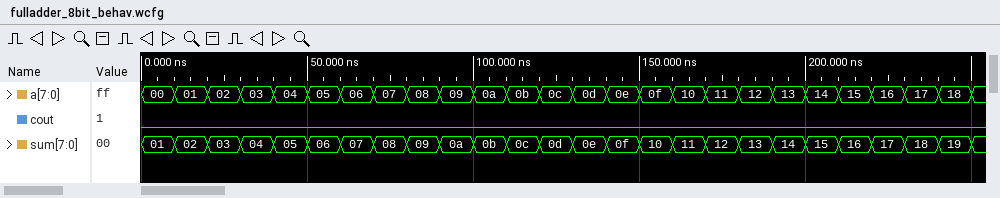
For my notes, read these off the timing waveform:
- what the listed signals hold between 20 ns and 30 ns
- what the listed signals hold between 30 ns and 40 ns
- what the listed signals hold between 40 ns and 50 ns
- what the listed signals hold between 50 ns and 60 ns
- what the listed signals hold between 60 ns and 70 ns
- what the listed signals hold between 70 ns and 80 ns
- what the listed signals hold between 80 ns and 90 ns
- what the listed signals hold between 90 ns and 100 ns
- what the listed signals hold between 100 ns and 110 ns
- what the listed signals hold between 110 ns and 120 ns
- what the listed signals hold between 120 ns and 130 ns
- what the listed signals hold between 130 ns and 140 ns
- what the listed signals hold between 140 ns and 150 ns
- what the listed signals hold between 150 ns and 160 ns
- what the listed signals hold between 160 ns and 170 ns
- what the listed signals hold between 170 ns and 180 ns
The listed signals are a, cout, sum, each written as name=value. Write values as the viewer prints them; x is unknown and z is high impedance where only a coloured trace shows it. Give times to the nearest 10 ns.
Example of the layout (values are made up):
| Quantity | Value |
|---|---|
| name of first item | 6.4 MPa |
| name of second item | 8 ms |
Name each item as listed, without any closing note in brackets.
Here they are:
| Quantity | Value |
|---|---|
| what the listed signals hold between 20 ns and 30 ns | a=02, cout=0, sum=03 |
| what the listed signals hold between 30 ns and 40 ns | a=03, cout=0, sum=04 |
| what the listed signals hold between 40 ns and 50 ns | a=04, cout=0, sum=05 |
| what the listed signals hold between 50 ns and 60 ns | a=05, cout=0, sum=06 |
| what the listed signals hold between 60 ns and 70 ns | a=06, cout=0, sum=07 |
| what the listed signals hold between 70 ns and 80 ns | a=07, cout=0, sum=08 |
| what the listed signals hold between 80 ns and 90 ns | a=08, cout=0, sum=09 |
| what the listed signals hold between 90 ns and 100 ns | a=09, cout=0, sum=0a |
| what the listed signals hold between 100 ns and 110 ns | a=0a, cout=0, sum=0b |
| what the listed signals hold between 110 ns and 120 ns | a=0b, cout=0, sum=0c |
| what the listed signals hold between 120 ns and 130 ns | a=0c, cout=0, sum=0d |
| what the listed signals hold between 130 ns and 140 ns | a=0d, cout=0, sum=0e |
| what the listed signals hold between 140 ns and 150 ns | a=0e, cout=0, sum=0f |
| what the listed signals hold between 150 ns and 160 ns | a=0f, cout=0, sum=10 |
| what the listed signals hold between 160 ns and 170 ns | a=10, cout=0, sum=11 |
| what the listed signals hold between 170 ns and 180 ns | a=11, cout=0, sum=12 |
